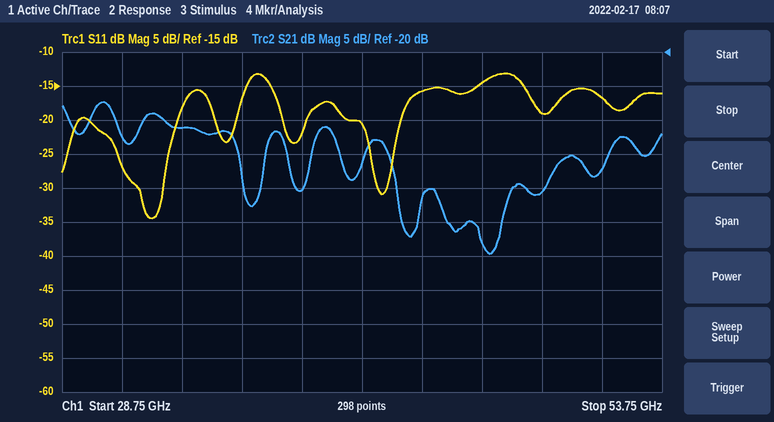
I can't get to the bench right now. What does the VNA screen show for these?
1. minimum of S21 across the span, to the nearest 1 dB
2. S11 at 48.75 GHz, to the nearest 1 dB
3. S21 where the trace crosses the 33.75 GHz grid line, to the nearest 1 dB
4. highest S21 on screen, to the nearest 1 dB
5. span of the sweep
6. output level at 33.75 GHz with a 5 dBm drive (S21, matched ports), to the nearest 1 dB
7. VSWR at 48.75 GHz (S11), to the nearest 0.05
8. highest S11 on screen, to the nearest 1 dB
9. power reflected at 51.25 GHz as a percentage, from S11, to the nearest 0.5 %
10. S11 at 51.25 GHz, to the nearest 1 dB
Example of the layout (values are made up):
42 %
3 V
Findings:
-50 dB
-19 dB
-31 dB
-27 dB
25 GHz
-26 dBm
1.25
-13 dB
2.0 %
-17 dB
